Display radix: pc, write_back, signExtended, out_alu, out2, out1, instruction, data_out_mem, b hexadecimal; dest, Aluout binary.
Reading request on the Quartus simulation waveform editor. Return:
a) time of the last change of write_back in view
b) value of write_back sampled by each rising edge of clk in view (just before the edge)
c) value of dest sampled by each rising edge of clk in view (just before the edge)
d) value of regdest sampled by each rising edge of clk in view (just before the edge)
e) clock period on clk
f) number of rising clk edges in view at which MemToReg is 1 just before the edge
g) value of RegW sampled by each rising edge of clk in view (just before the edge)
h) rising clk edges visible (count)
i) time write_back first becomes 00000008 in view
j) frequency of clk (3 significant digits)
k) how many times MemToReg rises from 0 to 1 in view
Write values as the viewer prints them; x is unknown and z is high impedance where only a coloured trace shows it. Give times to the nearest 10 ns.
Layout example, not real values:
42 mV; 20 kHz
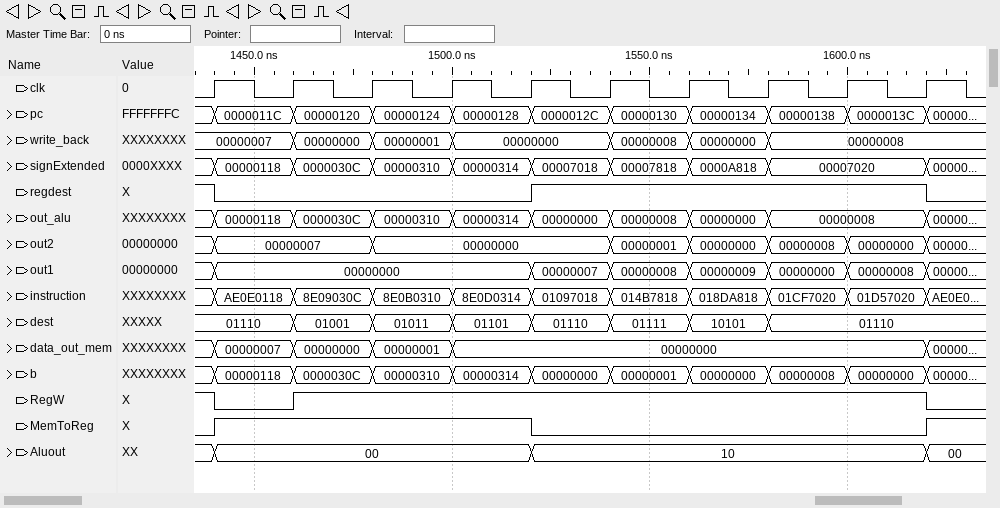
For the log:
1580 ns; 00000007, 00000007, 00000000, 00000001, 00000000, 00000000, 00000008, 00000000, 00000008, 00000008; 01110, 01110, 01001, 01011, 01101, 01110, 01111, 10101, 01110, 01110; 1 0 0 0 0 1 1 1 1 1; 20 ns; 4; 1 0 1 1 1 1 1 1 1 1; 10; 1540 ns; 50.0 MHz; 2
